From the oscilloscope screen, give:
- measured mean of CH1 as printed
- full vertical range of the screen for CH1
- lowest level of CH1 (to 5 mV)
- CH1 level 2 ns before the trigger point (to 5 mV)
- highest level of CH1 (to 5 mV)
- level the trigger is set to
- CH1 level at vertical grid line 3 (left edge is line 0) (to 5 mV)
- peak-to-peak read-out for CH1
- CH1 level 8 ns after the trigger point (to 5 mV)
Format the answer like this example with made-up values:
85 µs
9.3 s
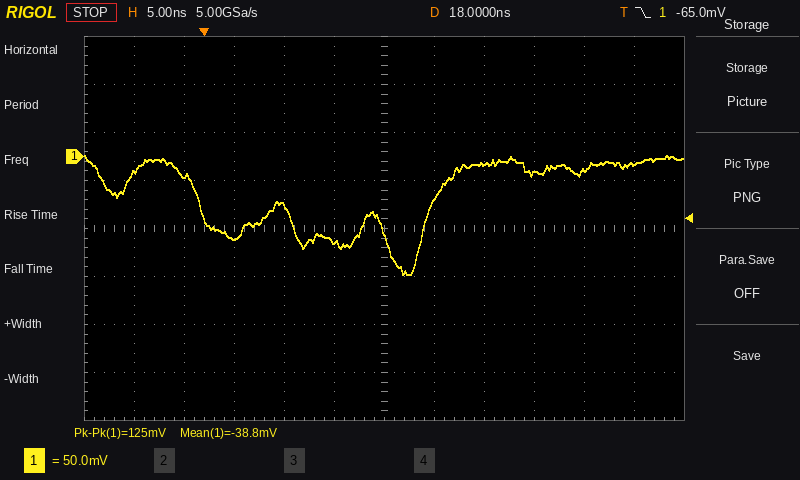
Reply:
-38.8 mV
400 mV
-125 mV
-20 mV
0 mV
-65.0 mV
-85 mV
125 mV
-50 mV
